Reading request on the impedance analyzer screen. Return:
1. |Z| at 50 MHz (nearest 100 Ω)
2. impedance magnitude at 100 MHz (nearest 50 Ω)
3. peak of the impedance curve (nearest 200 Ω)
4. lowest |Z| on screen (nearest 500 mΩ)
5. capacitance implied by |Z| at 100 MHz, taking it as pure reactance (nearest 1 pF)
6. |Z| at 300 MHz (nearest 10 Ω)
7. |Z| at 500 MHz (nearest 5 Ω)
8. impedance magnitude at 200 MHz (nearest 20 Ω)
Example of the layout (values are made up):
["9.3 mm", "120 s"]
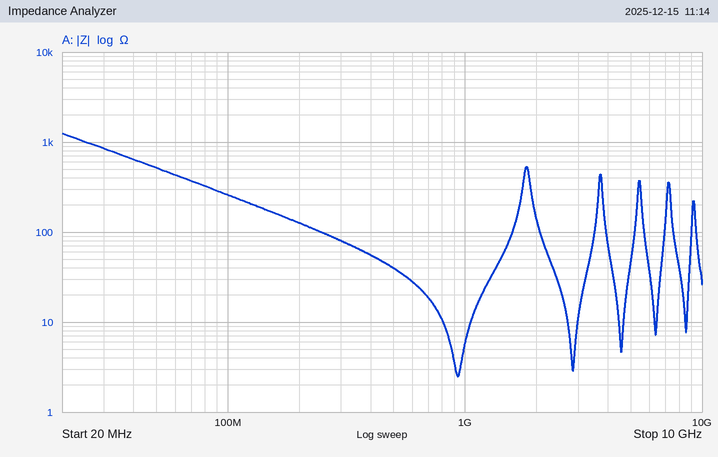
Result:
["500 Ω", "250 Ω", "1.2 kΩ", "2.5 Ω", "6 pF", "80 Ω", "40 Ω", "120 Ω"]
